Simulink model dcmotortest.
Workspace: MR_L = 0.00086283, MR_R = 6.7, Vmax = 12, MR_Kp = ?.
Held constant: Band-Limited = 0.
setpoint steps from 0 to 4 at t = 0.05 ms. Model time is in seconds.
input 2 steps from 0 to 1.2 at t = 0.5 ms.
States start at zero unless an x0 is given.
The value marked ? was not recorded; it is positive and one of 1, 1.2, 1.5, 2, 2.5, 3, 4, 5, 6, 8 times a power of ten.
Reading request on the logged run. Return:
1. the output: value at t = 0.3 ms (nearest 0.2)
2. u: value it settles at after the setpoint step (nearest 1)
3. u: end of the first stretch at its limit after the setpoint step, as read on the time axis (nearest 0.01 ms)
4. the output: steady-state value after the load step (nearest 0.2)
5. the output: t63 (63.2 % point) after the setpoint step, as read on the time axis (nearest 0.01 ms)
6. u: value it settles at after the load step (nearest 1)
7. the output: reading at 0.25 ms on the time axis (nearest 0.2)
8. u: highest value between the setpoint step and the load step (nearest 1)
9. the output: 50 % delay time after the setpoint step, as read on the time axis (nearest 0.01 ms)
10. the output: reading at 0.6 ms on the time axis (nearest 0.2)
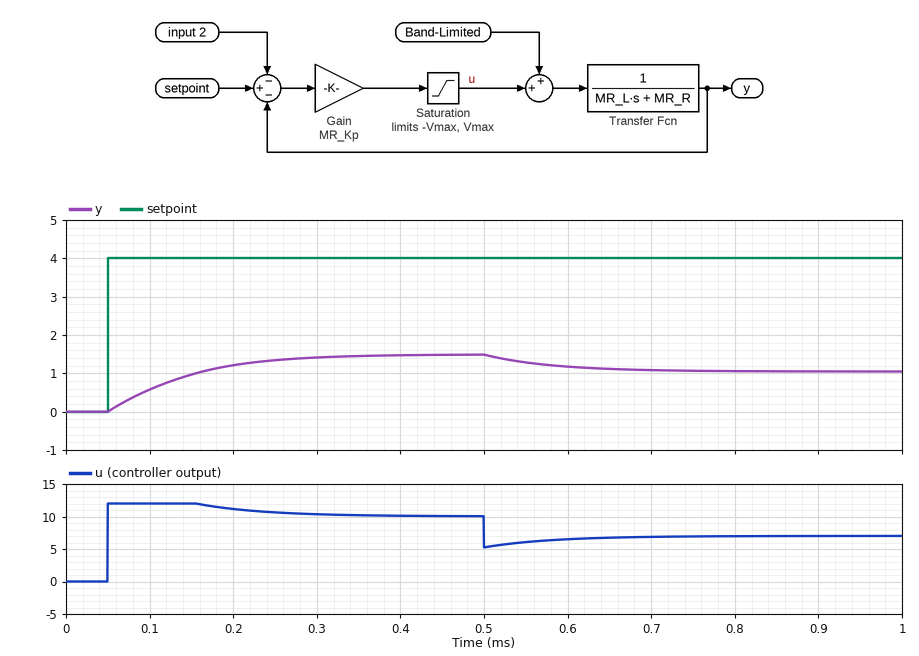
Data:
1.4
10
0.16 ms
1.0
0.15 ms
7
1.4
12
0.12 ms
1.2
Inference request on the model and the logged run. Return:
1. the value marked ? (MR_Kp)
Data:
4
